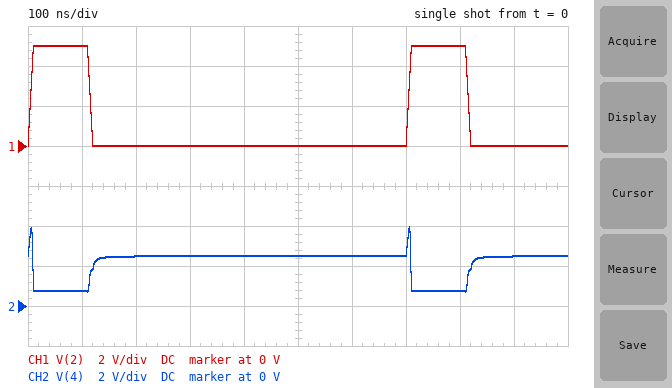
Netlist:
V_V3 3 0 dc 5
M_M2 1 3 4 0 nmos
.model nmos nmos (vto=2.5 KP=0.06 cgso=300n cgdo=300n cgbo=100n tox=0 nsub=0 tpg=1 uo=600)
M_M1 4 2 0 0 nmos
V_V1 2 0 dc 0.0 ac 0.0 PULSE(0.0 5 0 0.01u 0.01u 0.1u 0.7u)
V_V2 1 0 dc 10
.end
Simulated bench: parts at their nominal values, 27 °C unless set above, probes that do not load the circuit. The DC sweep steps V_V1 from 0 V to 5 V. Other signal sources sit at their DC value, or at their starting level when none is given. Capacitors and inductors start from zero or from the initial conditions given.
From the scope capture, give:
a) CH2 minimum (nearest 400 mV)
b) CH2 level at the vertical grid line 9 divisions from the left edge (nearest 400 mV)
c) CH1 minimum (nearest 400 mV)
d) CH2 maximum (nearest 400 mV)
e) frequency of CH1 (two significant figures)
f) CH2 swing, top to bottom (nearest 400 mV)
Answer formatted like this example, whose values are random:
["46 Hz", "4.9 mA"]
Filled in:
["800 mV", "2.4 V", "0 V", "4.0 V", "1.4 MHz", "3.2 V"]
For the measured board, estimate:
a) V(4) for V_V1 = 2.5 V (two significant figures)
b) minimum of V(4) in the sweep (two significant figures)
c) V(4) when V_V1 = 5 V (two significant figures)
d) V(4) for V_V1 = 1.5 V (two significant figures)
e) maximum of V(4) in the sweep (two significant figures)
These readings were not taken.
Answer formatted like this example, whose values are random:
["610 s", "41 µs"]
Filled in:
["2.5 V", "730 mV", "730 mV", "2.5 V", "2.5 V"]
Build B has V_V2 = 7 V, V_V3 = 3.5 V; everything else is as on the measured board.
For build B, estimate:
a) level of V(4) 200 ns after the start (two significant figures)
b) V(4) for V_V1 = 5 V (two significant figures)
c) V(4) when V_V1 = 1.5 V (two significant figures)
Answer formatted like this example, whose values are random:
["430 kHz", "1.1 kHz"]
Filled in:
["980 mV", "150 mV", "1.0 V"]
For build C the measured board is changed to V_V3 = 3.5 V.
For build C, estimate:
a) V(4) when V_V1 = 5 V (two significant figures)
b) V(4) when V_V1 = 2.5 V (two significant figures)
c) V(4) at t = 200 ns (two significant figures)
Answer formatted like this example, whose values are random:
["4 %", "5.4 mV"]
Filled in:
["150 mV", "1.0 V", "980 mV"]
